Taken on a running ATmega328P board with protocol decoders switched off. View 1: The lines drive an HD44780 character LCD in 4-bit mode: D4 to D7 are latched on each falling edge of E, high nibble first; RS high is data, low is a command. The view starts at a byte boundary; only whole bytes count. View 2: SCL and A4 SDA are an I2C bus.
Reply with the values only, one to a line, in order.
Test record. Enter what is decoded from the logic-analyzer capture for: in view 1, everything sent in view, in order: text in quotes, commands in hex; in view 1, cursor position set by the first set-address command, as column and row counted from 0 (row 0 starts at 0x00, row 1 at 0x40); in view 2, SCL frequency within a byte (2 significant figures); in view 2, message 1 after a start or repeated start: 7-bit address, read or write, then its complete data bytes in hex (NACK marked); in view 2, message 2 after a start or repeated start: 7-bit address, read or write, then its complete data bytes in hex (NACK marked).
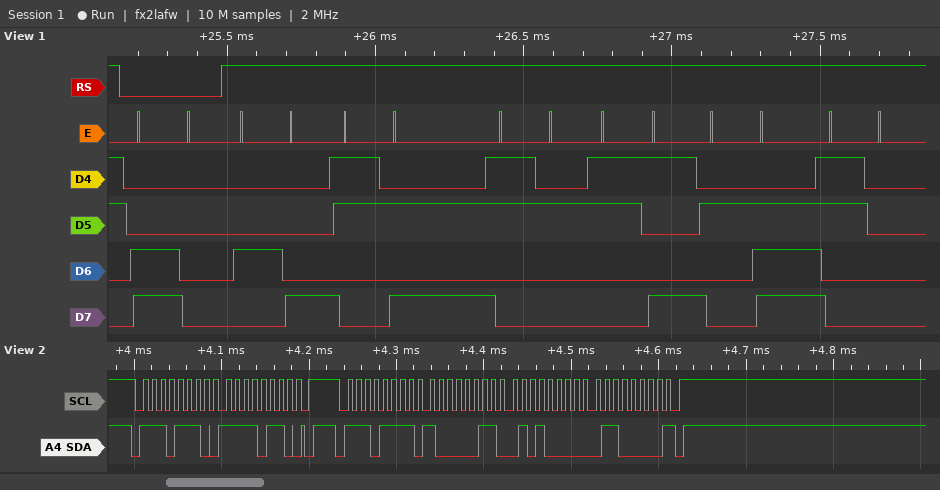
0xC0 "H:29.0"
column 0, row 1
100 kHz
0x77 write: F6
0x77 read: 83 50 60 NACK
